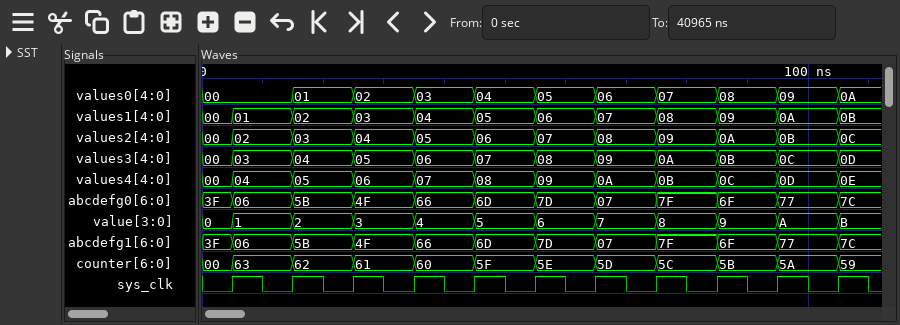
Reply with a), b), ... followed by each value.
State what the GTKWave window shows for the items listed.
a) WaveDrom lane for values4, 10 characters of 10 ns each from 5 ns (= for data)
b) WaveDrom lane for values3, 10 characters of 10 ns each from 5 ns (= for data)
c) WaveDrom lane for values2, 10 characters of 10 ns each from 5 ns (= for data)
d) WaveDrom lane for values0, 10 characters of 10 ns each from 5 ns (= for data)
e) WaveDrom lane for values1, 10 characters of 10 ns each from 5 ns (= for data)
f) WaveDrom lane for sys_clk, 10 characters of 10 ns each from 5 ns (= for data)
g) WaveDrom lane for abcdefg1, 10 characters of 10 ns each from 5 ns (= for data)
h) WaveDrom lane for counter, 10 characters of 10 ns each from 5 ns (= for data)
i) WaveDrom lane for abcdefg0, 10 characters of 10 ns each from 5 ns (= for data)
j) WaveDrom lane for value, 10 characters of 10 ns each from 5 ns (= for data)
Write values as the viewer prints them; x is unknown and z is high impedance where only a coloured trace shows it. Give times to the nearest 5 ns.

a) {name: 'values4', wave: '==========', data: '04 05 06 07 08 09 0A 0B 0C 0D'}
b) {name: 'values3', wave: '==========', data: '03 04 05 06 07 08 09 0A 0B 0C'}
c) {name: 'values2', wave: '==========', data: '02 03 04 05 06 07 08 09 0A 0B'}
d) {name: 'values0', wave: '==========', data: '00 01 02 03 04 05 06 07 08 09'}
e) {name: 'values1', wave: '==========', data: '01 02 03 04 05 06 07 08 09 0A'}
f) {name: 'sys_clk', wave: 'p.........'}
g) {name: 'abcdefg1', wave: '==========', data: '06 5B 4F 66 6D 7D 07 7F 6F 77'}
h) {name: 'counter', wave: '==========', data: '63 62 61 60 5F 5E 5D 5C 5B 5A'}
i) {name: 'abcdefg0', wave: '==========', data: '06 5B 4F 66 6D 7D 07 7F 6F 77'}
j) {name: 'value', wave: '==========', data: '1 2 3 4 5 6 7 8 9 A'}
